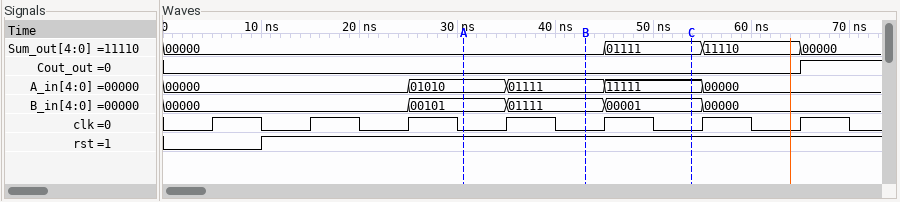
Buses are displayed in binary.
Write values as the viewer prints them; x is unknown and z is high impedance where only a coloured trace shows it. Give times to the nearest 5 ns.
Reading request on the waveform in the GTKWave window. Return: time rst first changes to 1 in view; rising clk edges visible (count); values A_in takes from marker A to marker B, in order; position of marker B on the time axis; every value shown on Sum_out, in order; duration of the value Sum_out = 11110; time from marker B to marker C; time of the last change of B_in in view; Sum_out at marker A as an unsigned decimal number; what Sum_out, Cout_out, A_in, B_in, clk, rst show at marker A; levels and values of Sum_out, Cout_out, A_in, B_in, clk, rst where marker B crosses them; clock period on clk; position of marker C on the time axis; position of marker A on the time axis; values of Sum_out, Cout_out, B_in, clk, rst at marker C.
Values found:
10 ns
7
01010, 01111
45 ns
00000, 01111, 11110, 00000
10 ns
10 ns
55 ns
0
Sum_out=00000, Cout_out=0, A_in=01010, B_in=00101, clk=0, rst=1
Sum_out=00000, Cout_out=0, A_in=01111, B_in=01111, clk=0, rst=1
10 ns
55 ns
30 ns
Sum_out=01111, Cout_out=0, B_in=00001, clk=0, rst=1
